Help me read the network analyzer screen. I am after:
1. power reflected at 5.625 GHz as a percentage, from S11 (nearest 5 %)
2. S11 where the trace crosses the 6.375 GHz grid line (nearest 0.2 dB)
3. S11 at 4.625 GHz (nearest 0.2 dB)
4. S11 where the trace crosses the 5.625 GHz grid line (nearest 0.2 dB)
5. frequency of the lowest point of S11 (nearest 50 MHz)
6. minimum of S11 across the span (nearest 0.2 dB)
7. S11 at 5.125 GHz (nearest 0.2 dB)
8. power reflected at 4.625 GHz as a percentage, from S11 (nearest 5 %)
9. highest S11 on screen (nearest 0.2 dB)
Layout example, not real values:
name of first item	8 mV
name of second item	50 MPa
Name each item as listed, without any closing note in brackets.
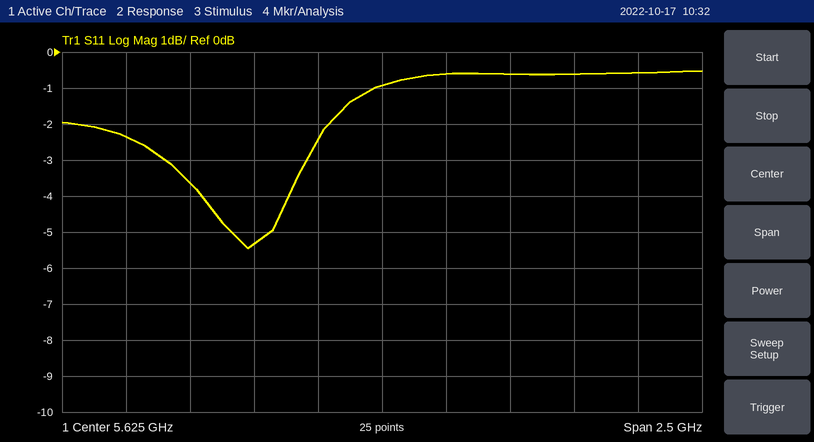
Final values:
power reflected at 5.625 GHz as a percentage, from S11	80 %
S11 where the trace crosses the 6.375 GHz grid line	-0.6 dB
S11 at 4.625 GHz	-2.4 dB
S11 where the trace crosses the 5.625 GHz grid line	-1.0 dB
frequency of the lowest point of S11	5.10 GHz
minimum of S11 across the span	-5.4 dB
S11 at 5.125 GHz	-5.4 dB
power reflected at 4.625 GHz as a percentage, from S11	60 %
highest S11 on screen	-0.6 dB
